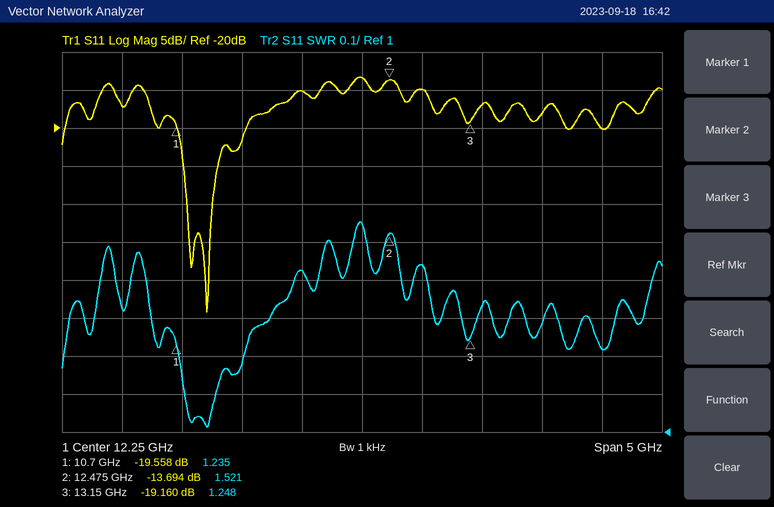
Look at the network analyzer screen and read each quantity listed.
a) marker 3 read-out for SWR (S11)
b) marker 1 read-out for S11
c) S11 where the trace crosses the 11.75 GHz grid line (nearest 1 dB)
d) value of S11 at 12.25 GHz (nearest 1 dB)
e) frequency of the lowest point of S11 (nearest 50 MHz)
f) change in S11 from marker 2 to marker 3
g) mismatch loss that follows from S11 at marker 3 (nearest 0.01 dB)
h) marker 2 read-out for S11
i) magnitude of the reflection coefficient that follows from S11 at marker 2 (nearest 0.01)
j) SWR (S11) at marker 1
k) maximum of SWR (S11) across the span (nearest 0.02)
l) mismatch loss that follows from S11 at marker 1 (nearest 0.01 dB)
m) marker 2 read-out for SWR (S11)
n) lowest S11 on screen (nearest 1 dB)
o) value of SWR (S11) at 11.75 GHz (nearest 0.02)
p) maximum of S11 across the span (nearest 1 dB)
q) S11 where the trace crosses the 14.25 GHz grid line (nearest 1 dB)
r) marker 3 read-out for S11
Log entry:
1.248
-19.558 dB
-15 dB
-13 dB
10.95 GHz
-5.466 dB
0.05 dB
-13.694 dB
0.21
1.235
1.56
0.05 dB
1.521
-44 dB
1.42
-13 dB
-20 dB
-19.160 dB
